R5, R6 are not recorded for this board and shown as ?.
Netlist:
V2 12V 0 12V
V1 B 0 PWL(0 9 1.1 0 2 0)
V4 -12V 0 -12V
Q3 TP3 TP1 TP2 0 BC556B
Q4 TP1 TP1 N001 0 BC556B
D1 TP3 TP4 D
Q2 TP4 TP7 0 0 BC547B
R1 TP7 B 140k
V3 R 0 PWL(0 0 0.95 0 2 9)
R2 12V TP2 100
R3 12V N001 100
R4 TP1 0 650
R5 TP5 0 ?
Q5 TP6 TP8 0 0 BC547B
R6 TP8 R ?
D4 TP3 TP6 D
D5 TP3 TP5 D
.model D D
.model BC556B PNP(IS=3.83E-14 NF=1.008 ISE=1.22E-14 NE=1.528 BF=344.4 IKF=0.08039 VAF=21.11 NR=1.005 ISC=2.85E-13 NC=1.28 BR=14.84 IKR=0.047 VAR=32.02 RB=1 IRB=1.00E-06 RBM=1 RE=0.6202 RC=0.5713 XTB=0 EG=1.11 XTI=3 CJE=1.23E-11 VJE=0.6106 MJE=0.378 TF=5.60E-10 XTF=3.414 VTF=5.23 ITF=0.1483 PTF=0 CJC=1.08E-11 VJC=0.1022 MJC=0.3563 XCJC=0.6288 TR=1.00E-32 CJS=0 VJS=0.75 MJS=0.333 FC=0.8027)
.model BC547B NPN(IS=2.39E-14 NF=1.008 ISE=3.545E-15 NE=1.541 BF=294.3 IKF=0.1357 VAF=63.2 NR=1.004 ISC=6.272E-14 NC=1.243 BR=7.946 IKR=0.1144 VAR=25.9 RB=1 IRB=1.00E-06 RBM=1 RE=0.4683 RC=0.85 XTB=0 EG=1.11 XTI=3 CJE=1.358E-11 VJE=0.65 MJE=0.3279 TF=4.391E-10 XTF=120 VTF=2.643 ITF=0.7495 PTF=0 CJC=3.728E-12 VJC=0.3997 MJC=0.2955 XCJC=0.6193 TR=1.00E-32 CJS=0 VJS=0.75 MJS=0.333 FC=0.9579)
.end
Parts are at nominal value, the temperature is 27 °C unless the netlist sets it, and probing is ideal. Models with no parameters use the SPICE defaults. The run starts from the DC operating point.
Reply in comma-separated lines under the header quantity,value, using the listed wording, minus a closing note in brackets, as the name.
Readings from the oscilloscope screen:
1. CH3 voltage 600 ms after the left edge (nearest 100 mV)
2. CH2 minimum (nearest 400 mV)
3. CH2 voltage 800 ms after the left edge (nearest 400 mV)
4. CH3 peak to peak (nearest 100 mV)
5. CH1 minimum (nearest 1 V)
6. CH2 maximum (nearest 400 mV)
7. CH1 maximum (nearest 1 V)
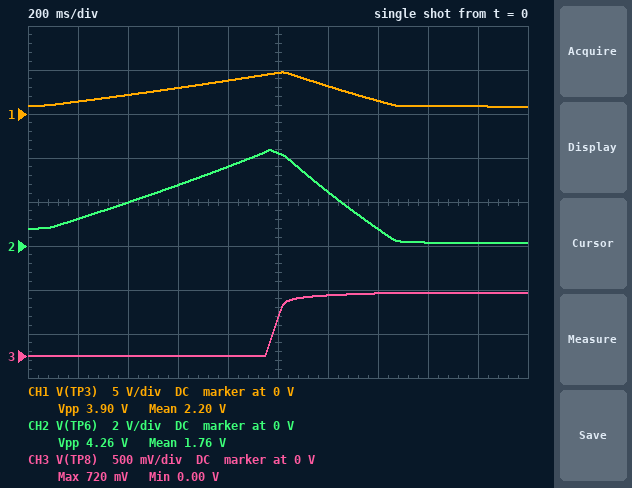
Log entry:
quantity,value
CH3 voltage 600 ms after the left edge,0 V
CH2 minimum,0 V
CH2 voltage 800 ms after the left edge,3.6 V
CH3 peak to peak,700 mV
CH1 minimum,1 V
CH2 maximum,4.4 V
CH1 maximum,5 V
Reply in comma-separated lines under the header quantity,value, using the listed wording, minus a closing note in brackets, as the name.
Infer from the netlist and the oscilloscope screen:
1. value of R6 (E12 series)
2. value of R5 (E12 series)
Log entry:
quantity,value
value of R6,68 kΩ
value of R5,270 Ω
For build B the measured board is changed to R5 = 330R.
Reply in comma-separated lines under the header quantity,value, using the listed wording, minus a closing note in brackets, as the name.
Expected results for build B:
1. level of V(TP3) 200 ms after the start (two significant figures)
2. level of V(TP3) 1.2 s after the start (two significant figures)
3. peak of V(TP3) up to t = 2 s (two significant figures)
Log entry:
quantity,value
level of V(TP3) 200 ms after the start,1.6 V
level of V(TP3) 1.2 s after the start,3.7 V
peak of V(TP3) up to t = 2 s,5.6 V
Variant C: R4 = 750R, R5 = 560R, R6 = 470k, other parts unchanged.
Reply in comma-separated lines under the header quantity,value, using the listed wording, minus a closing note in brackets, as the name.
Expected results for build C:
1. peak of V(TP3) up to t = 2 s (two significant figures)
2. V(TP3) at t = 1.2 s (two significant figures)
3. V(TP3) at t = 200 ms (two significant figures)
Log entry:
quantity,value
peak of V(TP3) up to t = 2 s,8.1 V
V(TP3) at t = 1.2 s,7.6 V
V(TP3) at t = 200 ms,1.2 V
